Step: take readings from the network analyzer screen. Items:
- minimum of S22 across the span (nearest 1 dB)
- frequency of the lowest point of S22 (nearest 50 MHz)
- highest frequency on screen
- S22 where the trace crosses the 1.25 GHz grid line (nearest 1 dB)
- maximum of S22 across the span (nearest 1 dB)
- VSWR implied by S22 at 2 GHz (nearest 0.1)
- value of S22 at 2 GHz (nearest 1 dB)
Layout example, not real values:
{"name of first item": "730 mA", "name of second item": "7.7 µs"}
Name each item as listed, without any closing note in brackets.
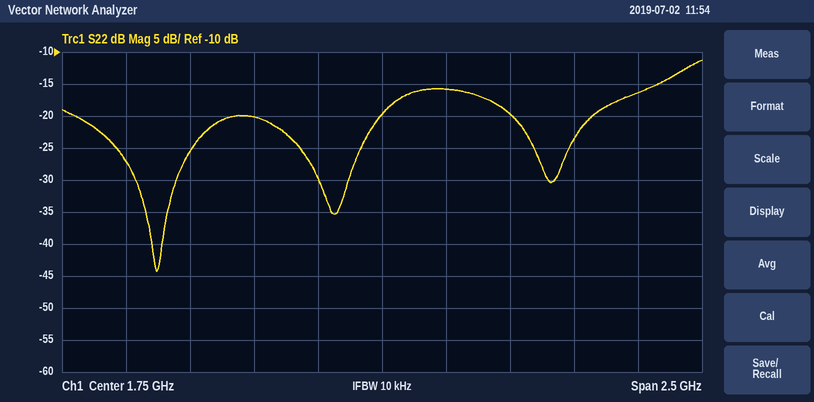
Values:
{"minimum of S22 across the span": "-44 dB", "frequency of the lowest point of S22": "850 MHz", "highest frequency on screen": "3 GHz", "S22 where the trace crosses the 1.25 GHz grid line": "-20 dB", "maximum of S22 across the span": "-11 dB", "VSWR implied by S22 at 2 GHz": "1.4", "value of S22 at 2 GHz": "-16 dB"}
